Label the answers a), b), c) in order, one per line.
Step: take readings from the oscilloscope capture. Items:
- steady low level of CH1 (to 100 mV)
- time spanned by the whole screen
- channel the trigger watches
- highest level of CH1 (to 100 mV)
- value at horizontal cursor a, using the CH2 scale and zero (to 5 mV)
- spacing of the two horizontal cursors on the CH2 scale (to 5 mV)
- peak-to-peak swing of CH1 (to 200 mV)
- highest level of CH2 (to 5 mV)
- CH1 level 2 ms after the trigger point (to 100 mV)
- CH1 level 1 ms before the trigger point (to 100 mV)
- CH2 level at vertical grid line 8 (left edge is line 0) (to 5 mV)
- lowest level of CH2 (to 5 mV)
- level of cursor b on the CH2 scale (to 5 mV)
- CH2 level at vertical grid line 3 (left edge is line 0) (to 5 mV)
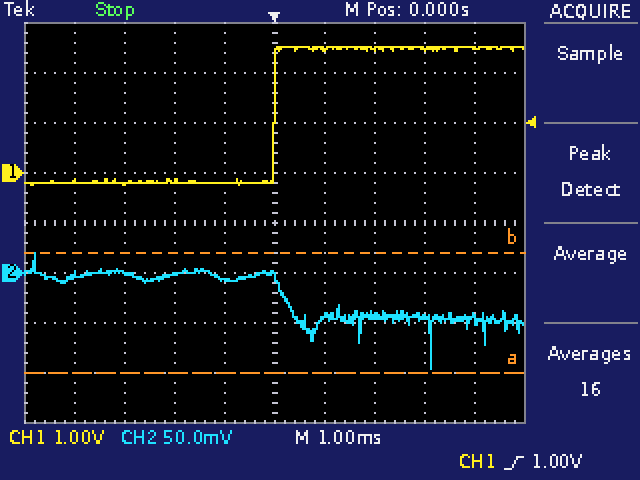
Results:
a) -200 mV
b) 10 ms
c) CH1
d) 2.5 V
e) -100 mV
f) 120 mV
g) 2.8 V
h) 20 mV
i) 2.5 V
j) -200 mV
k) -45 mV
l) -95 mV
m) 20 mV
n) 0 mV
